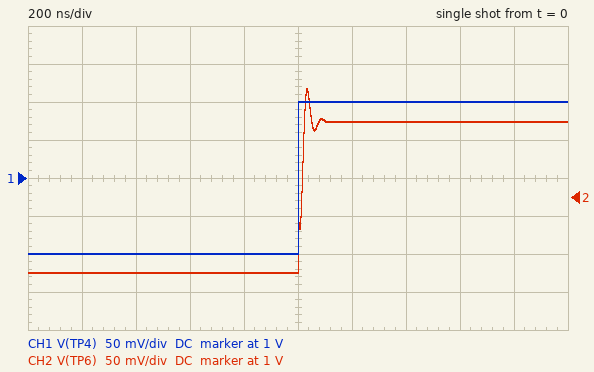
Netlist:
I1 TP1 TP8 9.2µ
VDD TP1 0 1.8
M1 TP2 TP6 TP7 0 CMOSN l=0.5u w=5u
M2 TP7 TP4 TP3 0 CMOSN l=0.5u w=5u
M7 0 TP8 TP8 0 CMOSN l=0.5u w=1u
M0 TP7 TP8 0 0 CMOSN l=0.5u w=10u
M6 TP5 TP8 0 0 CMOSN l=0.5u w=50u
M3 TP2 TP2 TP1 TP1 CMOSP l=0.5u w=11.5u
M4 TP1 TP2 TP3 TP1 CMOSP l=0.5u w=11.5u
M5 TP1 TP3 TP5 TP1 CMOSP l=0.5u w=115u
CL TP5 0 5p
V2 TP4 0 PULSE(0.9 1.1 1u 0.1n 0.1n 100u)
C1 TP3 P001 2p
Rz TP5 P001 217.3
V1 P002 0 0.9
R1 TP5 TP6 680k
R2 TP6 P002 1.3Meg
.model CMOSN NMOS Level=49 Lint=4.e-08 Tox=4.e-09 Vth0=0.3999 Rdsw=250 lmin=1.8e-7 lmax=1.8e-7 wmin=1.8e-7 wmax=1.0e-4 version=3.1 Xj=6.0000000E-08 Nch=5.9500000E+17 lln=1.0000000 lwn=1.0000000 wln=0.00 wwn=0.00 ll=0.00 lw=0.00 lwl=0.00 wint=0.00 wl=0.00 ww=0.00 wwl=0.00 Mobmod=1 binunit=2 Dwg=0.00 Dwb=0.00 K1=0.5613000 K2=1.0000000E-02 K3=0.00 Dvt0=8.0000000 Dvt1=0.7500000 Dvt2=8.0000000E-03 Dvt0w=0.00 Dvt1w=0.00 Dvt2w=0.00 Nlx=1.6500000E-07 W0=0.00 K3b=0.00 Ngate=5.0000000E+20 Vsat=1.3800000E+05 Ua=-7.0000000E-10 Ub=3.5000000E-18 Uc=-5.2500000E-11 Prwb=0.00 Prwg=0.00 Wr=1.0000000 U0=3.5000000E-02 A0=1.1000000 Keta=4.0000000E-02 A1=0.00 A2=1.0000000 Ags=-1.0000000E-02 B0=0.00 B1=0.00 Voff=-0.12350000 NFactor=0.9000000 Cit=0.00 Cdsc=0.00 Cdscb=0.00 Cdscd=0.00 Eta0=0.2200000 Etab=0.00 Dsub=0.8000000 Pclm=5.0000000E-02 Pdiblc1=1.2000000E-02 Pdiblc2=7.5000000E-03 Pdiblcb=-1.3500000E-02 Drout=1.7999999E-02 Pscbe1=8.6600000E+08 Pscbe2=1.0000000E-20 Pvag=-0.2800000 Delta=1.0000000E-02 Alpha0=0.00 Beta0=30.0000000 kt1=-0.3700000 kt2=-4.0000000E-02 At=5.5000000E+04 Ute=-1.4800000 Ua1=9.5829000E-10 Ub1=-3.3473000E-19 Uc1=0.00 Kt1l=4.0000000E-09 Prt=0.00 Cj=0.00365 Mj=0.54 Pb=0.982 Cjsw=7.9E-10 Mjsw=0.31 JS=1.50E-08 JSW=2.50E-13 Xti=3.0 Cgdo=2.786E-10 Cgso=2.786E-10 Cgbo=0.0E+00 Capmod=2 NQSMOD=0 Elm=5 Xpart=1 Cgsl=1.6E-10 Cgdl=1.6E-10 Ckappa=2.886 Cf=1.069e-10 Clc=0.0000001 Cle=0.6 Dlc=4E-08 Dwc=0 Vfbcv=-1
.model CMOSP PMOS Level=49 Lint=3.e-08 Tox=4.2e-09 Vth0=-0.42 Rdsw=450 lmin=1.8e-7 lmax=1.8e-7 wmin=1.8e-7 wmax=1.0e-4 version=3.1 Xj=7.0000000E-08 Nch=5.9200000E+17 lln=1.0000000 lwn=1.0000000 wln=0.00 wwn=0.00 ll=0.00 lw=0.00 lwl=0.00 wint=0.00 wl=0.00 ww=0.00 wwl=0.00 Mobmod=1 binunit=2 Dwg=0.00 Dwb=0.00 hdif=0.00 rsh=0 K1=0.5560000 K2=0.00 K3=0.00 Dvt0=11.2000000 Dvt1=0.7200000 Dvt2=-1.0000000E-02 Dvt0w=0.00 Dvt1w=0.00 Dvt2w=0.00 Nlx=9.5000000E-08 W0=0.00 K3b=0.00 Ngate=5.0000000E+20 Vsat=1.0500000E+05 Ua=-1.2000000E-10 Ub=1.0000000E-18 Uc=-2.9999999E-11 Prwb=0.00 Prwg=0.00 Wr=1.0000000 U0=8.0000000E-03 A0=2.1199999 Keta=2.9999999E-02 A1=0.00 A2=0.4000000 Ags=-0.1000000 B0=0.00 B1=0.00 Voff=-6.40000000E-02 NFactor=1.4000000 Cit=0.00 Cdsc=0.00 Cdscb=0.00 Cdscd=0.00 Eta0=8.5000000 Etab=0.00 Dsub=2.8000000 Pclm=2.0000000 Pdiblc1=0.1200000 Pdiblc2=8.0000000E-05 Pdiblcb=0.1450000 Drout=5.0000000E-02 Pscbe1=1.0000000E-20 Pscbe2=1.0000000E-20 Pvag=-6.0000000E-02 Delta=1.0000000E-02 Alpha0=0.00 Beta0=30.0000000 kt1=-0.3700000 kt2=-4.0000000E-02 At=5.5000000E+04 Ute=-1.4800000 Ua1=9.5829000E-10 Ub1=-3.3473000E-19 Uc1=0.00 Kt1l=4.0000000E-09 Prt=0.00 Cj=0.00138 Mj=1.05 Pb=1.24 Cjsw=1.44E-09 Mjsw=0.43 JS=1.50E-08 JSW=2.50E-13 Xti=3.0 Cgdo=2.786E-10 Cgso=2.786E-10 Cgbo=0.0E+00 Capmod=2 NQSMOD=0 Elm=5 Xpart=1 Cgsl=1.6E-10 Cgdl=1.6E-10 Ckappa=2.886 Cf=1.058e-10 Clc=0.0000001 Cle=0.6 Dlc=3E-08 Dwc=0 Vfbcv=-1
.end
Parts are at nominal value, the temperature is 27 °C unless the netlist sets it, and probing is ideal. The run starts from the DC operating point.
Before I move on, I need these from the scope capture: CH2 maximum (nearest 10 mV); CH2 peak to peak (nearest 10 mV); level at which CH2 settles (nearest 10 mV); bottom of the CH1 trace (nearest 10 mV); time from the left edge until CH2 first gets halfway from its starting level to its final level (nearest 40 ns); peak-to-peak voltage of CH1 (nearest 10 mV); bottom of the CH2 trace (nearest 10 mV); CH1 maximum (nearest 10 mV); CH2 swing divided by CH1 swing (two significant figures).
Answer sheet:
1.14 V
240 mV
1.10 V
900 mV
1.00 µs
200 mV
900 mV
1.10 V
1.2
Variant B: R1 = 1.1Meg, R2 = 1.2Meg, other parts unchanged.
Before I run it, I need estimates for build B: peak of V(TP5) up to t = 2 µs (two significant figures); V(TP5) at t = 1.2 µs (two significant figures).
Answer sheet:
1.4 V
1.3 V
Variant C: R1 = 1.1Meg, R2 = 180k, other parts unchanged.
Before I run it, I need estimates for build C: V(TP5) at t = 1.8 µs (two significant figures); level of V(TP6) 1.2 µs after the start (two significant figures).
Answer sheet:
1.8 V
1.0 V
